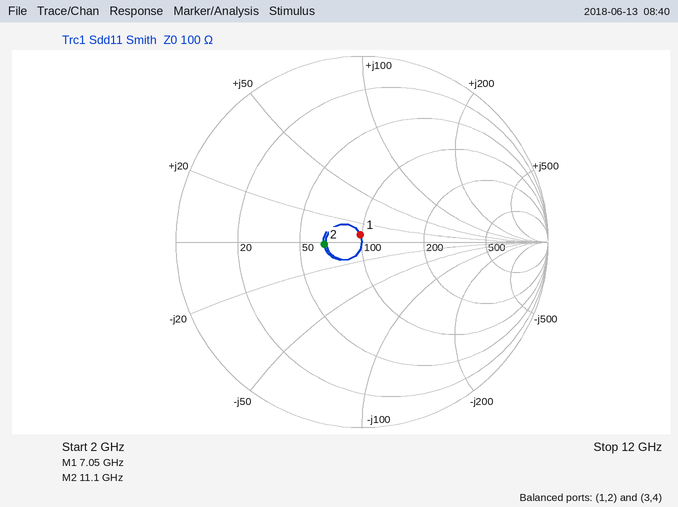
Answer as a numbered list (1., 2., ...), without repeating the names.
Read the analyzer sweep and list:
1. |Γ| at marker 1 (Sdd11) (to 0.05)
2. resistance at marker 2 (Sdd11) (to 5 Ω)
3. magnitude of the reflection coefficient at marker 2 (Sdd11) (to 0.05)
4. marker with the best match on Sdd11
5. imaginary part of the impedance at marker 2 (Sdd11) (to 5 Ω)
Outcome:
1. 0.05
2. 65 Ω
3. 0.20
4. marker 1
5. 0 Ω
